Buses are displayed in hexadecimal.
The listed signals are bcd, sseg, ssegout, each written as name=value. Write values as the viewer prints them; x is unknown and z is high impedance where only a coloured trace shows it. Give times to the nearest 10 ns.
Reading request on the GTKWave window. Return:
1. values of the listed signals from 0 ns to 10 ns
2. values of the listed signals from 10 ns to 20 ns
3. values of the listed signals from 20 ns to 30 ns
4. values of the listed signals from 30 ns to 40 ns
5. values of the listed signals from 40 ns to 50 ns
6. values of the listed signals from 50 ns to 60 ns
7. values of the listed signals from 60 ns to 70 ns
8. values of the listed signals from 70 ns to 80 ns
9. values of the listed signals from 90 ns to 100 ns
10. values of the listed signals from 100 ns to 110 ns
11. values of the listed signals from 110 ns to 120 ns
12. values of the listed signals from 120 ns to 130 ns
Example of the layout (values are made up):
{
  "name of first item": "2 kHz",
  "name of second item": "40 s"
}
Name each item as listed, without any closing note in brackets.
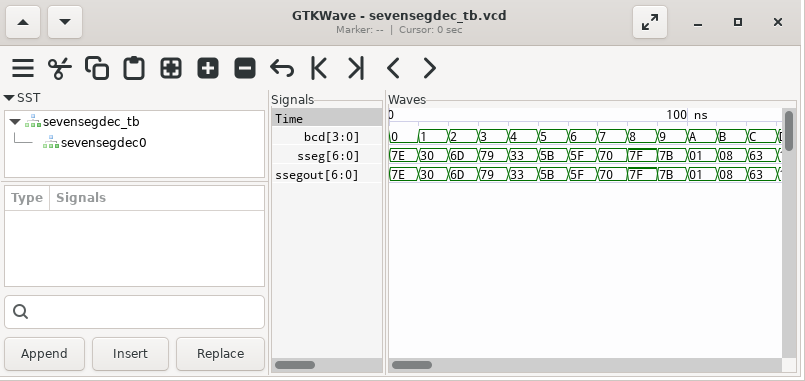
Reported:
{
  "values of the listed signals from 0 ns to 10 ns": "bcd=0, sseg=7E, ssegout=7E",
  "values of the listed signals from 10 ns to 20 ns": "bcd=1, sseg=30, ssegout=30",
  "values of the listed signals from 20 ns to 30 ns": "bcd=2, sseg=6D, ssegout=6D",
  "values of the listed signals from 30 ns to 40 ns": "bcd=3, sseg=79, ssegout=79",
  "values of the listed signals from 40 ns to 50 ns": "bcd=4, sseg=33, ssegout=33",
  "values of the listed signals from 50 ns to 60 ns": "bcd=5, sseg=5B, ssegout=5B",
  "values of the listed signals from 60 ns to 70 ns": "bcd=6, sseg=5F, ssegout=5F",
  "values of the listed signals from 70 ns to 80 ns": "bcd=7, sseg=70, ssegout=70",
  "values of the listed signals from 90 ns to 100 ns": "bcd=9, sseg=7B, ssegout=7B",
  "values of the listed signals from 100 ns to 110 ns": "bcd=A, sseg=01, ssegout=01",
  "values of the listed signals from 110 ns to 120 ns": "bcd=B, sseg=08, ssegout=08",
  "values of the listed signals from 120 ns to 130 ns": "bcd=C, sseg=63, ssegout=63"
}
